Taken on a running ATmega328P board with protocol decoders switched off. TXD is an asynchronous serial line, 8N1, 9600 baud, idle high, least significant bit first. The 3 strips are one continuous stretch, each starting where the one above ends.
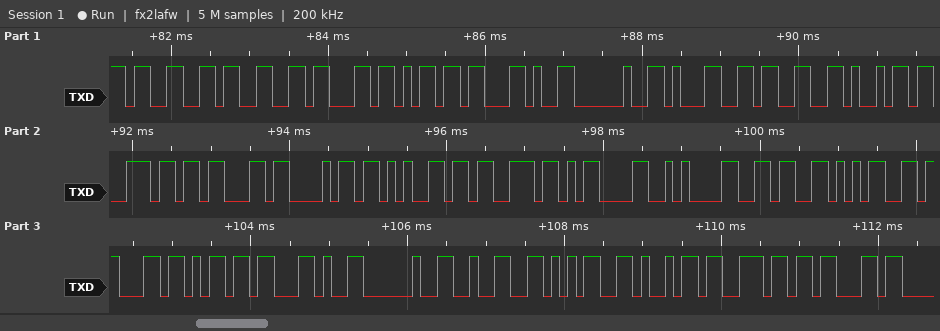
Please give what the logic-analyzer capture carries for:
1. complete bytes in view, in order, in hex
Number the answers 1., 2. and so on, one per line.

1. 33 33 63 6D 2C 20 31 33 69 6E 63 68 65 73 0D 0A 36 35 63 6D 2C 20 32 35 69 6E 63
